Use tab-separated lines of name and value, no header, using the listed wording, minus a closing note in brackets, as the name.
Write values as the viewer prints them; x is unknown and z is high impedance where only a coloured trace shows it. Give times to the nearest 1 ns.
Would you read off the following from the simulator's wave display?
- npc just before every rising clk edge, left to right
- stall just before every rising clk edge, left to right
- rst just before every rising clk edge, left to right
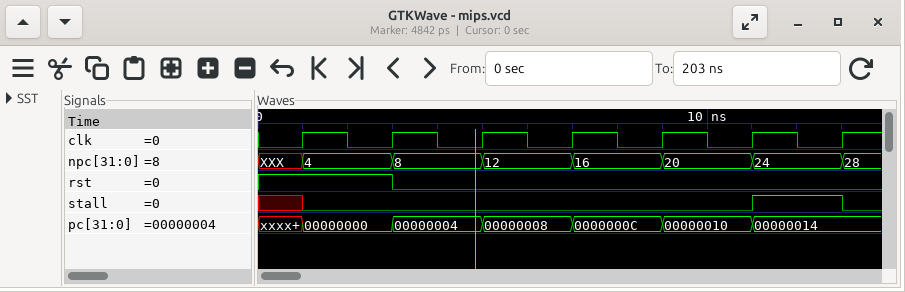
npc just before every rising clk edge, left to right	XXX, 4, 8, 12, 16, 20, 24
stall just before every rising clk edge, left to right	x 0 0 0 0 0 1
rst just before every rising clk edge, left to right	1 1 0 0 0 0 0
